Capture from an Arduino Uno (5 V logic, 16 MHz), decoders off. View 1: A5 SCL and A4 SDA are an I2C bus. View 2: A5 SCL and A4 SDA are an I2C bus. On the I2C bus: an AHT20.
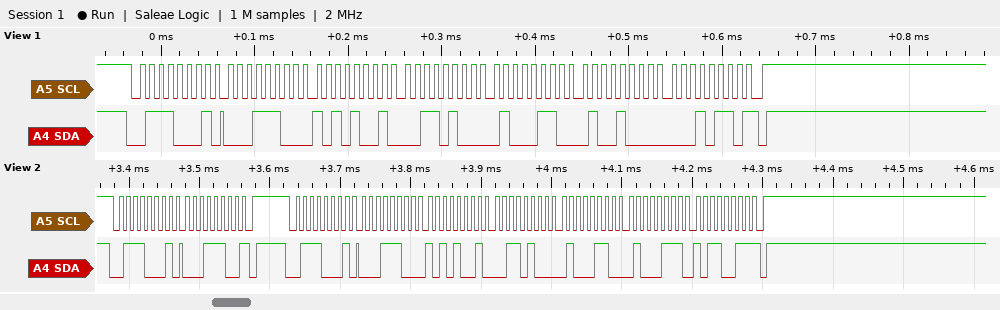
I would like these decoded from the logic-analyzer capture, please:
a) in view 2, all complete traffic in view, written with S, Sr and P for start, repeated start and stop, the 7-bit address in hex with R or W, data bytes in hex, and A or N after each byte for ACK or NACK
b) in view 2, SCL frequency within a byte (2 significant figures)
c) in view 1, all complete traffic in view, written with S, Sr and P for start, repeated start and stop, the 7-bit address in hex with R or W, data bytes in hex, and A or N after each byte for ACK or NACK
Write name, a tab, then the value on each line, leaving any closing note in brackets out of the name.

in view 2, all complete traffic in view, written with S, Sr and P for start, repeated start and stop, the 7-bit address in hex with R or W, data bytes in hex, and A or N after each byte for ACK or NACK	S 38R A 1C N P S 38R A 1C A A9 A 34 A 46 A 47 A B3 N P
in view 2, SCL frequency within a byte	100 kHz
in view 1, all complete traffic in view, written with S, Sr and P for start, repeated start and stop, the 7-bit address in hex with R or W, data bytes in hex, and A or N after each byte for ACK or NACK	S 38R A 1C A A9 A 34 A 46 A 48 A 16 N P
